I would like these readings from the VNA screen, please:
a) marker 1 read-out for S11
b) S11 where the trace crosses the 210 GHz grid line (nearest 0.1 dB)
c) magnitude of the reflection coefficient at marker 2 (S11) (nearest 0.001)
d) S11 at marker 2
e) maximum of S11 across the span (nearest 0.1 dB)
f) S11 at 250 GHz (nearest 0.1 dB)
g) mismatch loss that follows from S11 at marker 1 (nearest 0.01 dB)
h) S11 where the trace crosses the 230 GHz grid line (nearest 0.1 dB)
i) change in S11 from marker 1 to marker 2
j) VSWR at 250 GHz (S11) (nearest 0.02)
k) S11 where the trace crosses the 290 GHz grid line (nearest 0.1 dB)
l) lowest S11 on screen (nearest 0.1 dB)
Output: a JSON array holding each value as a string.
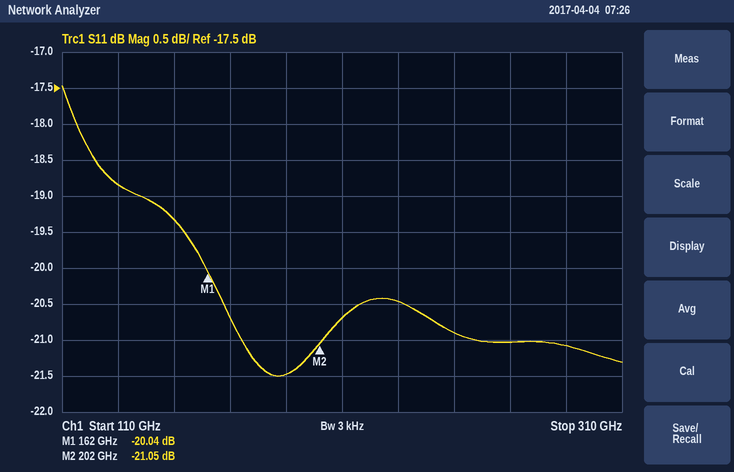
["-20.04 dB", "-20.7 dB", "0.089", "-21.05 dB", "-17.5 dB", "-20.9 dB", "0.04 dB", "-20.5 dB", "-1.01 dB", "1.20", "-21.1 dB", "-21.5 dB"]
